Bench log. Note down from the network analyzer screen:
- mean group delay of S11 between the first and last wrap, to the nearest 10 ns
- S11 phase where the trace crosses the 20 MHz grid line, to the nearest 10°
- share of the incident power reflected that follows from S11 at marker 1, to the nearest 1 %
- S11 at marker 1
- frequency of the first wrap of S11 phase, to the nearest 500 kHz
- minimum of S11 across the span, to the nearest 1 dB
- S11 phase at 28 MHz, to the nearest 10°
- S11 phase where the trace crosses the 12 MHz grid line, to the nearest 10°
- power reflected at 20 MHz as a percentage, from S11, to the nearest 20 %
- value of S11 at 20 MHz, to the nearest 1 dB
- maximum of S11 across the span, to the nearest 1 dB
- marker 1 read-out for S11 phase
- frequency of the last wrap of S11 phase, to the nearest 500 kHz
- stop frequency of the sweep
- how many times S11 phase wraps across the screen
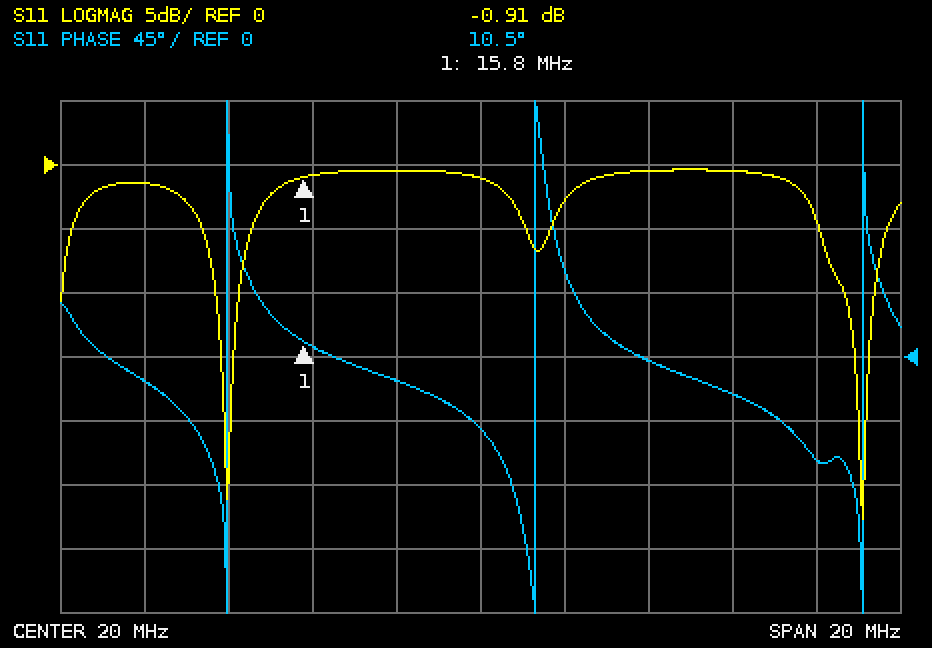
130 ns
-50°
81 %
-0.91 dB
14.0 MHz
-28 dB
-70°
-20°
80 %
-1 dB
0 dB
10.5°
29.0 MHz
30 MHz
3
